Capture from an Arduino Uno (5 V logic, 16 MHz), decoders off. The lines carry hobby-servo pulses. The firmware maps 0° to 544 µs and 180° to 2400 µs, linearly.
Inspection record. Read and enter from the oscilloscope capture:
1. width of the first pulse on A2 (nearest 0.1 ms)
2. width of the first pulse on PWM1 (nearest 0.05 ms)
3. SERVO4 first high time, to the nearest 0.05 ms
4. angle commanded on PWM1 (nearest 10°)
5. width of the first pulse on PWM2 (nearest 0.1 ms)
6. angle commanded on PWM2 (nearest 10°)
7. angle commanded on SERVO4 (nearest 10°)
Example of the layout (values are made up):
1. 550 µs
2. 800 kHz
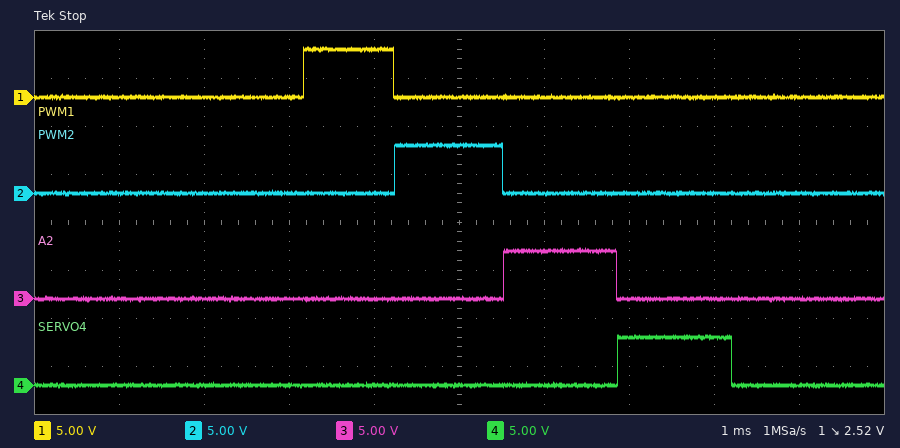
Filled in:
1. 1.3 ms
2. 1.05 ms
3. 1.35 ms
4. 50°
5. 1.3 ms
6. 70°
7. 80°
